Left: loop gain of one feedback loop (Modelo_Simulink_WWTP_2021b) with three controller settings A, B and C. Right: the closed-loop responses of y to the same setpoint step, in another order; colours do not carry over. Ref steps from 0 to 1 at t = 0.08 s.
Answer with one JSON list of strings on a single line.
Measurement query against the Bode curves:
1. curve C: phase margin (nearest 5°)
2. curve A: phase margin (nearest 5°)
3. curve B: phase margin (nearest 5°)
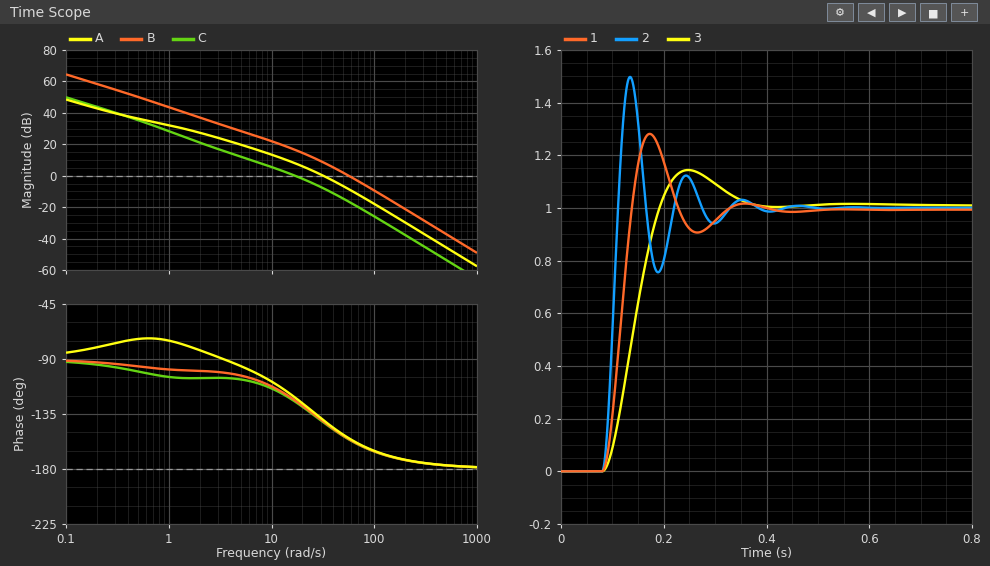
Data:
["55°", "40°", "25°"]
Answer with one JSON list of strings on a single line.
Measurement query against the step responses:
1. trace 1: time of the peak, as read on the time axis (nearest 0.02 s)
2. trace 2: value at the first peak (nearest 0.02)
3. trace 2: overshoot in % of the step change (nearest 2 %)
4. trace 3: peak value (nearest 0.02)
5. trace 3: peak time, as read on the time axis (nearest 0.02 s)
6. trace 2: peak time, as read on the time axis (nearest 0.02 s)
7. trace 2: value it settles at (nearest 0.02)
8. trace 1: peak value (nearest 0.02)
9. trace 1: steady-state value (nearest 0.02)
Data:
["0.18 s", "1.50", "50 %", "1.14", "0.24 s", "0.14 s", "1.00", "1.28", "1.00"]
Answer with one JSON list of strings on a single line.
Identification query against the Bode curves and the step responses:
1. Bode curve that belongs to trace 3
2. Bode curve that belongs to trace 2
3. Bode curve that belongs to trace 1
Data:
["C", "B", "A"]
